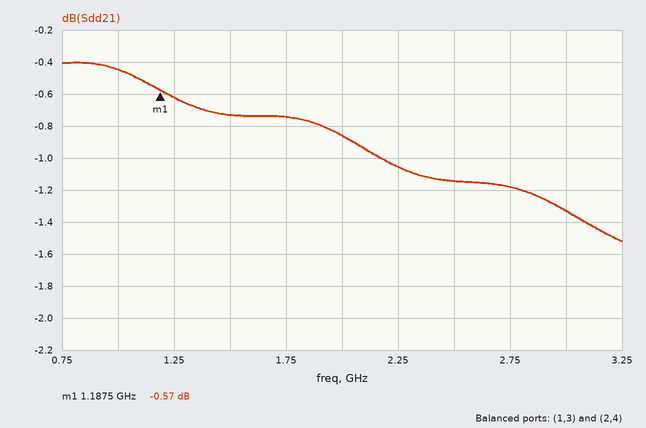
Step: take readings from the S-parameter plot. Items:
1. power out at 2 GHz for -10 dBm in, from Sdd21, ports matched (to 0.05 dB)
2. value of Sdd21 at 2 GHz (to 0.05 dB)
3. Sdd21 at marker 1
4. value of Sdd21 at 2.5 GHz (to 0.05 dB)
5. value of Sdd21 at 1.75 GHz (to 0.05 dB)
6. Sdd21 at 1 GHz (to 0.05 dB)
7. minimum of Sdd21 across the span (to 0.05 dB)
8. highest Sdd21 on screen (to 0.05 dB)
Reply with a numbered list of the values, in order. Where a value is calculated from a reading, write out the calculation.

1. -10 dBm + (-0.85 dB) = -10.85 dBm
2. -0.85 dB
3. -0.57 dB
4. -1.15 dB
5. -0.75 dB
6. -0.45 dB
7. -1.50 dB
8. -0.40 dB
